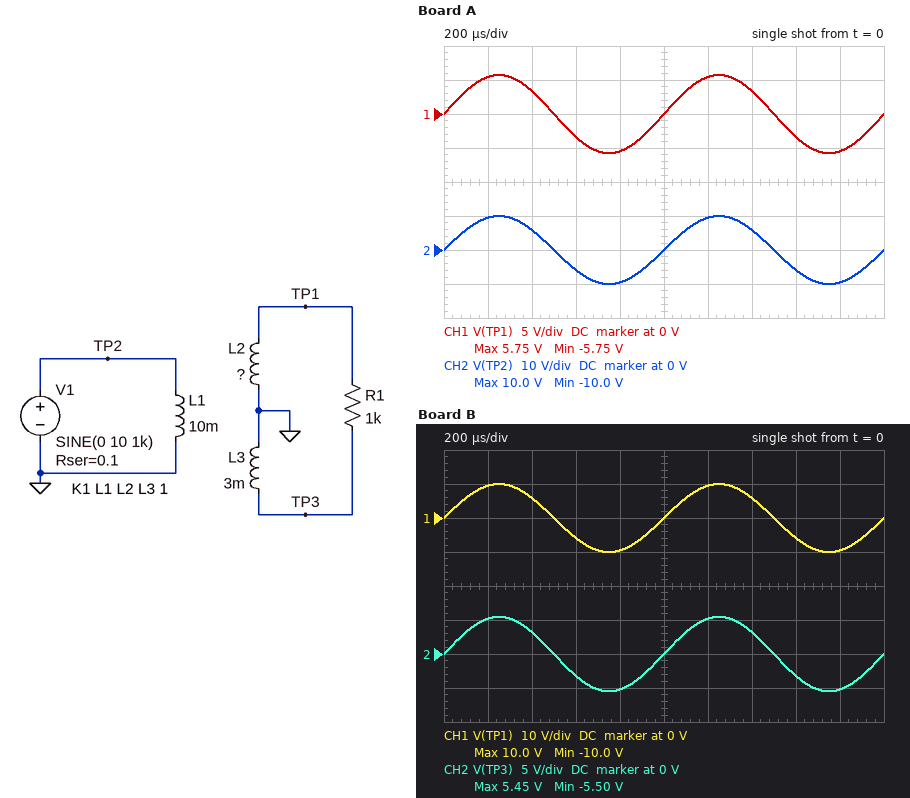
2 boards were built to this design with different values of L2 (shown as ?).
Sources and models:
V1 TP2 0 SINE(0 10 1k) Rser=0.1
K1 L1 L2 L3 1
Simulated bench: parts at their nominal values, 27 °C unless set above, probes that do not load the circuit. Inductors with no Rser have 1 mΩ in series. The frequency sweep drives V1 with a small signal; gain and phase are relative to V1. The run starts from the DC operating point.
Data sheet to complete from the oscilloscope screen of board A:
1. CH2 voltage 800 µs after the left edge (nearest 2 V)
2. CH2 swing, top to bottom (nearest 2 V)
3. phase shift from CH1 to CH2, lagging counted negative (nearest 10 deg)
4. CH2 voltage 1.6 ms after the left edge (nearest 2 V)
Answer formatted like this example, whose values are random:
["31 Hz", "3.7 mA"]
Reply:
["-10 V", "20 V", "0 deg", "-6 V"]
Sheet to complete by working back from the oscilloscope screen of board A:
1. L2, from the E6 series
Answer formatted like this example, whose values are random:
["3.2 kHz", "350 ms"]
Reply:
["3.3 mH"]
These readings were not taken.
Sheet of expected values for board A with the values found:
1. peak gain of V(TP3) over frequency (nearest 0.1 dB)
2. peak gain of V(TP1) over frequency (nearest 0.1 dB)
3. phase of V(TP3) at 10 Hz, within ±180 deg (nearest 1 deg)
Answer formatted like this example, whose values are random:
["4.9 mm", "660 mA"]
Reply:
["-5.2 dB", "-4.8 dB", "9 deg"]
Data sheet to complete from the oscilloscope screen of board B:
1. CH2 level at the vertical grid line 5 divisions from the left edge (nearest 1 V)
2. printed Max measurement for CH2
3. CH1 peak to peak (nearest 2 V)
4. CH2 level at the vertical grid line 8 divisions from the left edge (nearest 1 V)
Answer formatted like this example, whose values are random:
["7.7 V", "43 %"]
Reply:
["0 V", "5.45 V", "20 V", "-3 V"]
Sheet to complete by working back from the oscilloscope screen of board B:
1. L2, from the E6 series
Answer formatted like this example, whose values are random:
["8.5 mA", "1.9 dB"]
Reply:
["10 mH"]
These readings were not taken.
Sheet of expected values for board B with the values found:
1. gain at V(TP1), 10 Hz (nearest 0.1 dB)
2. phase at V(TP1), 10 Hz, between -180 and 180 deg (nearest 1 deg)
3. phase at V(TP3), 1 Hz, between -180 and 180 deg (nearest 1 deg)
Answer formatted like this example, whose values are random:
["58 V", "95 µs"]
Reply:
["-0.1 dB", "9 deg", "58 deg"]
